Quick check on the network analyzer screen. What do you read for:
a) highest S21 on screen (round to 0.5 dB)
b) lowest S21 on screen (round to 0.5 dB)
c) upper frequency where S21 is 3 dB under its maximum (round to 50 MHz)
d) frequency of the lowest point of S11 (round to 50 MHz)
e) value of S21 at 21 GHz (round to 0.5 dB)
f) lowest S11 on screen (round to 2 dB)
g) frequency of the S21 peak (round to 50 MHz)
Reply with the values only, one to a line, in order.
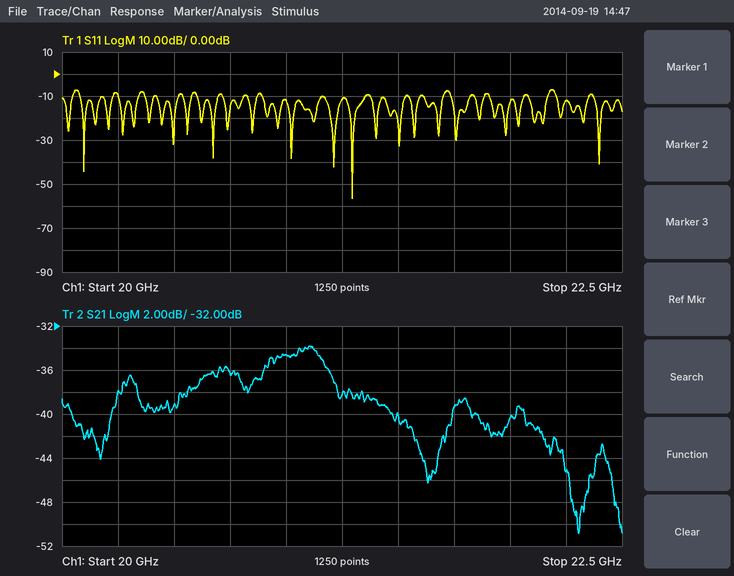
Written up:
-34.0 dB
-51.0 dB
21.20 GHz
21.30 GHz
-34.5 dB
-56 dB
21.10 GHz
